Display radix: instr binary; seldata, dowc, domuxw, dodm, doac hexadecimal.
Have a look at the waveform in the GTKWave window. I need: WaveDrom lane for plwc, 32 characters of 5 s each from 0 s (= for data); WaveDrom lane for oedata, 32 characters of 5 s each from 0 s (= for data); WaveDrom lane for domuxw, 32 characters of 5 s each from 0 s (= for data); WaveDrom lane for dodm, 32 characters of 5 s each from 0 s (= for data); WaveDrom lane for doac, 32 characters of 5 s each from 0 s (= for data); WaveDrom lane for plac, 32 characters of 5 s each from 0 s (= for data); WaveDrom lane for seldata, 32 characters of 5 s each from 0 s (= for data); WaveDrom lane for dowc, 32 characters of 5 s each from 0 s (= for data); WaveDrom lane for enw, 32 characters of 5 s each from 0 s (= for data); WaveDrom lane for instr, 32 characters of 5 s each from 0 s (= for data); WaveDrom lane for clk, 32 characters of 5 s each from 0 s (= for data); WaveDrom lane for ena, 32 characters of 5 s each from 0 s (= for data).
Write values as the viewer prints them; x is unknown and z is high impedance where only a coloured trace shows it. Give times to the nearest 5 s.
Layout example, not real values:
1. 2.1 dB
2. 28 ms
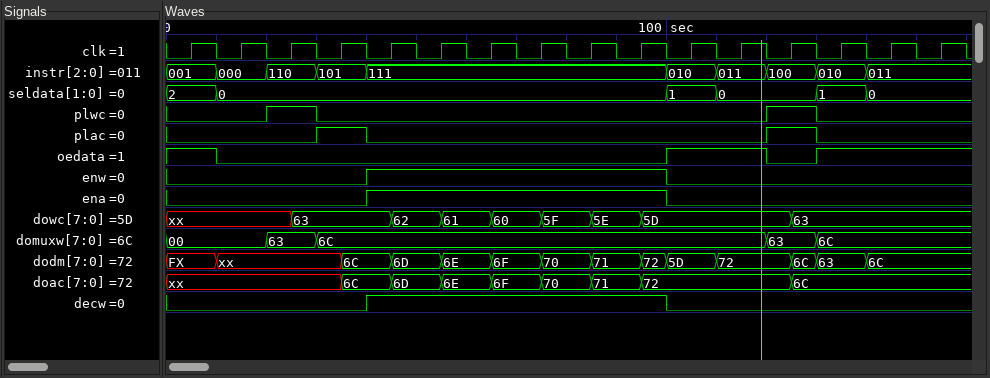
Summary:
1. {name: 'plwc', wave: '0...1.0.................1.0.....'}
2. {name: 'oedata', wave: '1.0.................1...0.1.....'}
3. {name: 'domuxw', wave: '=...=.=.................=.=.....', data: '00 63 6C 63 6C'}
4. {name: 'dodm', wave: '=.x....=.=.=.=.=.=.==.=..==.=...', data: 'FX 6C 6D 6E 6F 70 71 72 5D 72 6C 63 6C'}
5. {name: 'doac', wave: 'x......=.=.=.=.=.=.=.....=......', data: '6C 6D 6E 6F 70 71 72 6C'}
6. {name: 'plac', wave: '0.....1.0...............1.0.....'}
7. {name: 'seldata', wave: '=.=.................=.=...=.=...', data: '2 0 1 0 1 0'}
8. {name: 'dowc', wave: 'x....=...=.=.=.=.=.=.....=......', data: '63 62 61 60 5F 5E 5D 63'}
9. {name: 'enw', wave: '0.......1...........0...........'}
10. {name: 'instr', wave: '=.=.=.=.=...........=.=.=.=.=...', data: '001 000 110 101 111 010 011 100 010 011'}
11. {name: 'clk', wave: '01010101010101010101010101010101'}
12. {name: 'ena', wave: '0.......1...........0...........'}
